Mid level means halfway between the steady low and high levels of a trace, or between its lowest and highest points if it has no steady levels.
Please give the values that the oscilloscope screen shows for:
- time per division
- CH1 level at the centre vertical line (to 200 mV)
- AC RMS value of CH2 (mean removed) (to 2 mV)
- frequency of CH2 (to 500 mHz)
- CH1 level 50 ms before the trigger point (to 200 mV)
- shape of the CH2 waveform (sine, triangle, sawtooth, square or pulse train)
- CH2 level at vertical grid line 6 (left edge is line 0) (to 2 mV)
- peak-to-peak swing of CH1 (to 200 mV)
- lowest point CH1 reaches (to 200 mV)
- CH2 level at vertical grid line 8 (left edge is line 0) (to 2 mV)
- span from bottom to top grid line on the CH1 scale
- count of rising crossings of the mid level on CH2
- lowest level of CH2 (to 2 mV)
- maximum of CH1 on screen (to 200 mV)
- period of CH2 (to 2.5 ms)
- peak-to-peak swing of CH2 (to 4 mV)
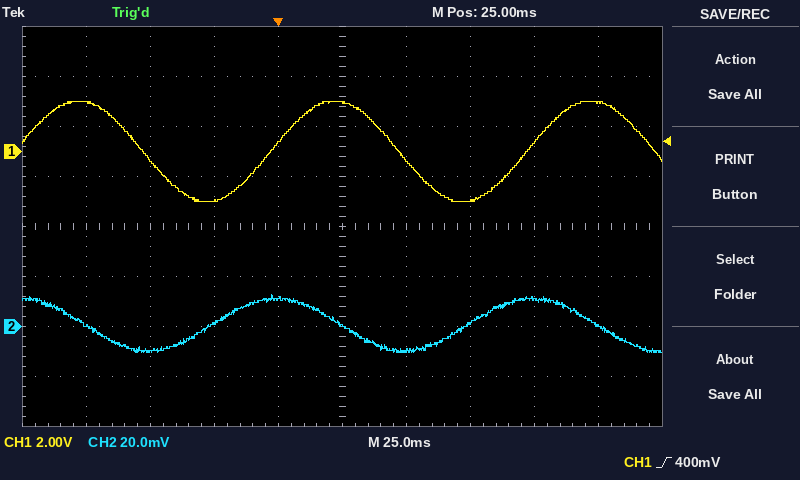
25 ms
2.0 V
8 mV
10.0 Hz
-400 mV
sine
-10 mV
4.0 V
-2.0 V
12 mV
16 V
2
-10 mV
2.0 V
100.0 ms
24 mV
